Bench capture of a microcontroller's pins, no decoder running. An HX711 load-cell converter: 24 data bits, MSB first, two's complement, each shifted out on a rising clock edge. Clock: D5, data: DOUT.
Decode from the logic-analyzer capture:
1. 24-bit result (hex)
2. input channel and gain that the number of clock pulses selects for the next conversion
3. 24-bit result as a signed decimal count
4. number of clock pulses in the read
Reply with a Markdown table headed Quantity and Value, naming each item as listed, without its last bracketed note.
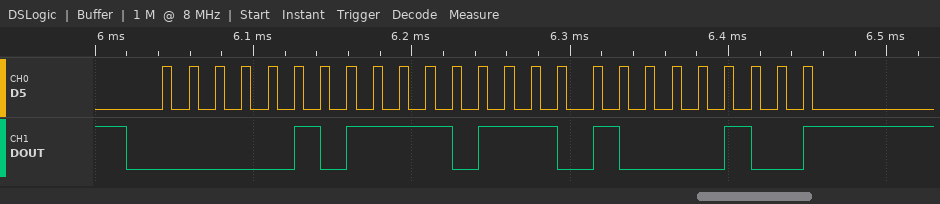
| Quantity | Value |
|---|---|
| 24-bit result | 0x05EE84 |
| input channel and gain that the number of clock pulses selects for the next conversion | channel A, gain 128 |
| 24-bit result as a signed decimal count | 388740 |
| number of clock pulses in the read | 25 |
